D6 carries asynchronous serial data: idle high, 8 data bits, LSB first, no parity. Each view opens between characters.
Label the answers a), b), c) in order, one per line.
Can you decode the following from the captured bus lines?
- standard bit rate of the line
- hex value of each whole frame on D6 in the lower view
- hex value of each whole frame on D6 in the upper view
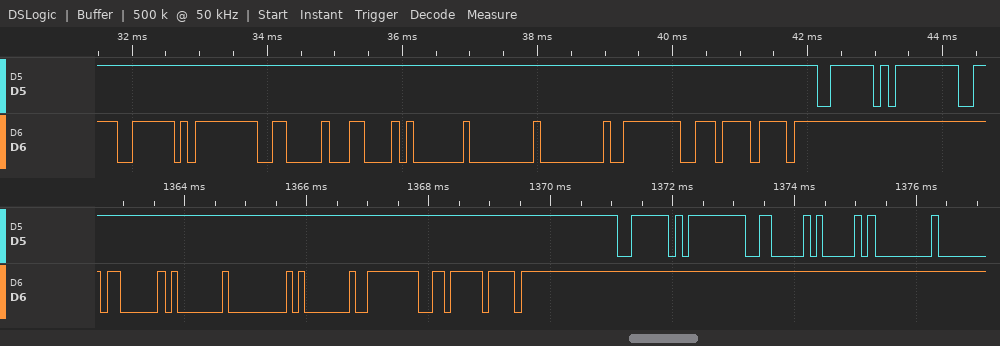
a) 9600 baud
b) 03, 01, 00, 01, FE, F6, EF
c) 7E, FF, 06, 0C, 01, 00, 00, FE, EE, EF
